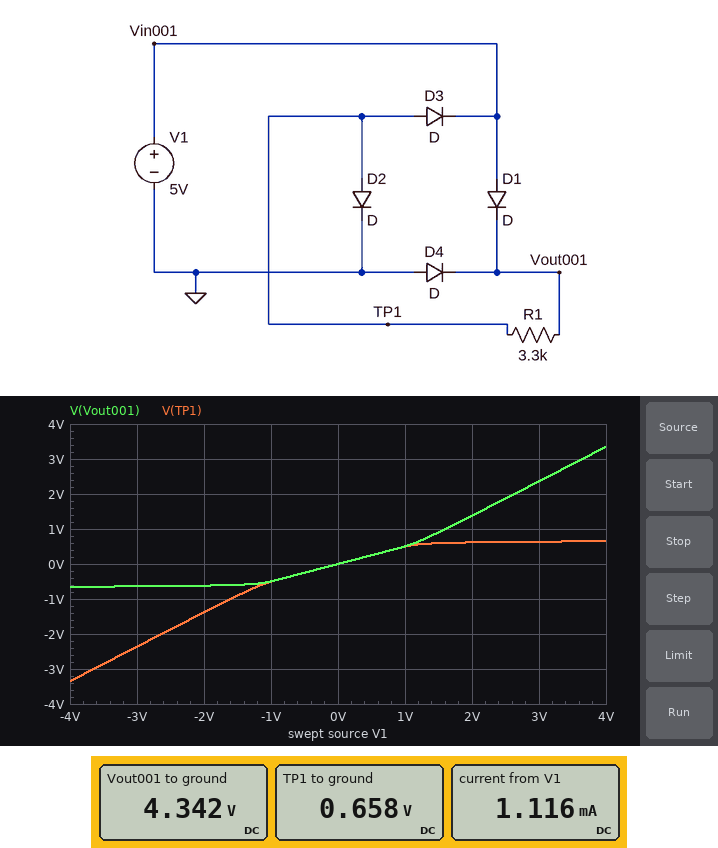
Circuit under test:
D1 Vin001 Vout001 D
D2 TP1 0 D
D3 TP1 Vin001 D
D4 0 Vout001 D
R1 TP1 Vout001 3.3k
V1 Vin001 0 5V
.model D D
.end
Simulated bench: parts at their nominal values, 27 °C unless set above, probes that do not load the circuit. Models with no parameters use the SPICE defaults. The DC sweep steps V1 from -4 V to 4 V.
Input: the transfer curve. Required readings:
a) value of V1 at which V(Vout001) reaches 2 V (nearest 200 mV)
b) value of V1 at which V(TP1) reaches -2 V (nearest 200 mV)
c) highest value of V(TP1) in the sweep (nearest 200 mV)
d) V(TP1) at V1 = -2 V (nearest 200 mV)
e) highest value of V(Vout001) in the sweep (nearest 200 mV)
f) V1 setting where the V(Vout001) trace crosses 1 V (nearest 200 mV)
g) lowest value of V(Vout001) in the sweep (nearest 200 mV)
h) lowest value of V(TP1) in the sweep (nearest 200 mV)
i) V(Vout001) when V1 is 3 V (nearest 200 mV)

2.6 V
-2.6 V
600 mV
-1.4 V
3.4 V
1.6 V
-600 mV
-3.4 V
2.4 V
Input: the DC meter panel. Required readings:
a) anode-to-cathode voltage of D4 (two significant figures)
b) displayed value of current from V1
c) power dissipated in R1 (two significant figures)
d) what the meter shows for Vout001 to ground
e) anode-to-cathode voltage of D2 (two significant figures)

-4.3 V
1.116 mA
4.1 mW
4.342 V
660 mV
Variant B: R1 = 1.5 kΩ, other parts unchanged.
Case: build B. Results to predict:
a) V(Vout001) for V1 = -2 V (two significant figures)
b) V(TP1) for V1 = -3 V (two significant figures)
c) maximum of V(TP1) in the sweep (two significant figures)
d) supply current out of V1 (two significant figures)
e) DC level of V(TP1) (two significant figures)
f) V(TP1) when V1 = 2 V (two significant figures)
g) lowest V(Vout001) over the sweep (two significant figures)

-640 mV
-2.3 V
670 mV
2.4 mA
680 mV
640 mV
-670 mV
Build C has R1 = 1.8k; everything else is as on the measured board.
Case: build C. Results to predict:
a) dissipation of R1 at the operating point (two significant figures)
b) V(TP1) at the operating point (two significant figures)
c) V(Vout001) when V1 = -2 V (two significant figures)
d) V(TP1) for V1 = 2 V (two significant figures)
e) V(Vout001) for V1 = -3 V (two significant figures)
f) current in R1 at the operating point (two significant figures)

7.4 mW
670 mV
-630 mV
630 mV
-650 mV
2.0 mA
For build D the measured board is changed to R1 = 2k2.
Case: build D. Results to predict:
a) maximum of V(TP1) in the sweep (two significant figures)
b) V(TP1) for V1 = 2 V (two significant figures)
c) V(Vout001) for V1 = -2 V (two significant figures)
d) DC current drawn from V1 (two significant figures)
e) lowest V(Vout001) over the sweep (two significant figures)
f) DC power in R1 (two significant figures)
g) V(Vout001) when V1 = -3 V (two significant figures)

660 mV
630 mV
-630 mV
1.7 mA
-660 mV
6.1 mW
-650 mV
